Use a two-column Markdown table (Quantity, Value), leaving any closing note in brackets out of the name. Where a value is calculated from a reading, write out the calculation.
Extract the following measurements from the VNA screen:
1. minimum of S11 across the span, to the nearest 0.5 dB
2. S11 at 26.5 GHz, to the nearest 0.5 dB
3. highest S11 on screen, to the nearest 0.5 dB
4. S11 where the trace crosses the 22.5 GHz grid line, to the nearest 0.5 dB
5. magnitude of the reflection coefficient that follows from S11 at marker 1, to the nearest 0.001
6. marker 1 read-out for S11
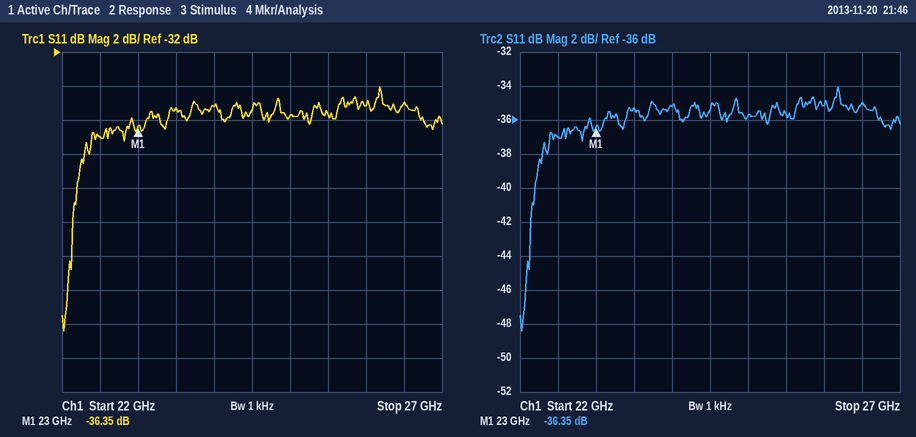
| Quantity | Value |
|---|---|
| minimum of S11 across the span, to the nearest 0.5 dB | -48.5 dB |
| S11 at 26.5 GHz, to the nearest 0.5 dB | -35.0 dB |
| highest S11 on screen, to the nearest 0.5 dB | -34.0 dB |
| S11 where the trace crosses the 22.5 GHz grid line, to the nearest 0.5 dB | -37.0 dB |
| magnitude of the reflection coefficient that follows from S11 at marker 1, to the nearest 0.001 | 10^(-36.35/20) ≈ 0.015 |
| marker 1 read-out for S11 | -36.35 dB |
